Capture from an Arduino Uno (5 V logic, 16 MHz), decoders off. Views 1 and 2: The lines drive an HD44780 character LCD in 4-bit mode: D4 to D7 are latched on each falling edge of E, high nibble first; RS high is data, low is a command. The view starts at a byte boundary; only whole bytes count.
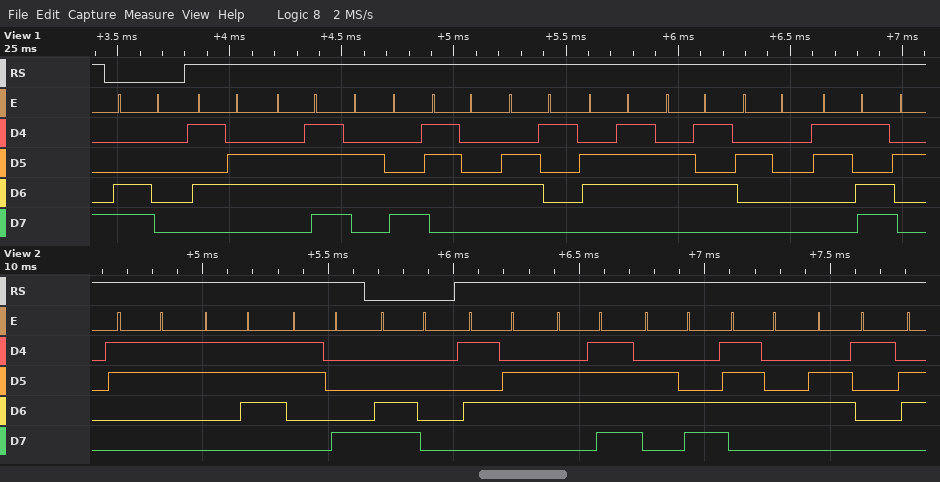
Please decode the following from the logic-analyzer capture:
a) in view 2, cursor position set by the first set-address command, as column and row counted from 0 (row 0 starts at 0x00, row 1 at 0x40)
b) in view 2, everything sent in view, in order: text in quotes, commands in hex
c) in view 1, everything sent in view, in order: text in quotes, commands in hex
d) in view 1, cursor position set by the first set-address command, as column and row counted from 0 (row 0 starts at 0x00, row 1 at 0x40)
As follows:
column 0, row 1
"378" 0xC0 "Volta"
0xC0 "Voltage ="
column 0, row 1
